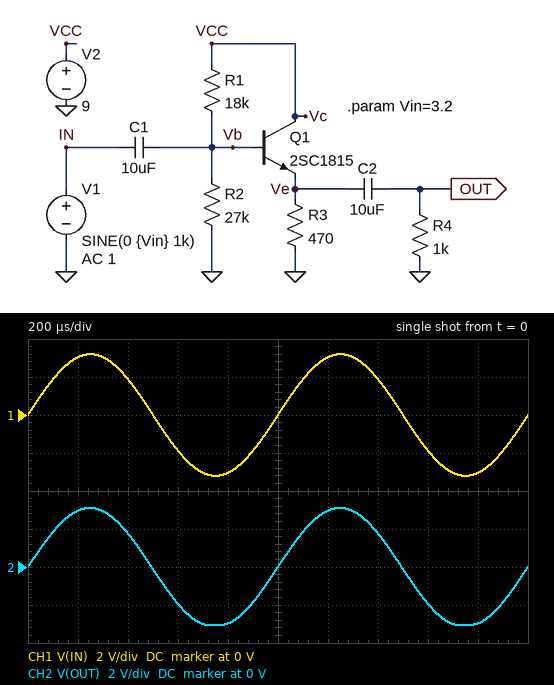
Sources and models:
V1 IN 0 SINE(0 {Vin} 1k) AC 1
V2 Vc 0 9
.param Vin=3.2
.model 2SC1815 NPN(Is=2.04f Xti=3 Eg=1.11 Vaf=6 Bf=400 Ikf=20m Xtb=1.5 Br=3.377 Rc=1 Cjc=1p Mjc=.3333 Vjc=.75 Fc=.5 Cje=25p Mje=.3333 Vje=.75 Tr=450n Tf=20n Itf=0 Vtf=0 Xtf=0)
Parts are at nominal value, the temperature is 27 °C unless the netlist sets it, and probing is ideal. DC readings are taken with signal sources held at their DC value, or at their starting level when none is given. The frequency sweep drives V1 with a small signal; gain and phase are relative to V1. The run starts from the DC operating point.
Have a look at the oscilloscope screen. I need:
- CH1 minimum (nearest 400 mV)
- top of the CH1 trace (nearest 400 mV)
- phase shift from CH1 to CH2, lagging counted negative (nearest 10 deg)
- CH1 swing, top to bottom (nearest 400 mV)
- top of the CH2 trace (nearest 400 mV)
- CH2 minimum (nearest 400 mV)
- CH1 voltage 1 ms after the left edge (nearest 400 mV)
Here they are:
-3.2 V
3.2 V
0 deg
6.4 V
3.2 V
-3.2 V
0 V
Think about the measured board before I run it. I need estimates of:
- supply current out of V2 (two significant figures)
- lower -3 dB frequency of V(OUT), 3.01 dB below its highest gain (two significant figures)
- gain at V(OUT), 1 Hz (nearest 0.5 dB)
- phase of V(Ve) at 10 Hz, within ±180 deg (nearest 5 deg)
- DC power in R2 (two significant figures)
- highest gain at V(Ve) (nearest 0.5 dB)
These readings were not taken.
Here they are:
9.7 mA
16 Hz
-29.5 dB
10 deg
1.0 mW
0 dB
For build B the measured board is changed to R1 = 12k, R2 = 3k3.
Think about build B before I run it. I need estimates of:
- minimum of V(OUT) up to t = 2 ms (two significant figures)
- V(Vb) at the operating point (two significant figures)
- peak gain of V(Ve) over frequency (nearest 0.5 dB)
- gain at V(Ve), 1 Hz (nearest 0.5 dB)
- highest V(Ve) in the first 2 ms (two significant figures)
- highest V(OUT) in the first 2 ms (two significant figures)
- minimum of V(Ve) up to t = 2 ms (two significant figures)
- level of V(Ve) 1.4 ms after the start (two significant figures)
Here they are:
-940 mV
1.9 V
-0.5 dB
-16.0 dB
4.4 V
3.1 V
410 mV
3.0 V
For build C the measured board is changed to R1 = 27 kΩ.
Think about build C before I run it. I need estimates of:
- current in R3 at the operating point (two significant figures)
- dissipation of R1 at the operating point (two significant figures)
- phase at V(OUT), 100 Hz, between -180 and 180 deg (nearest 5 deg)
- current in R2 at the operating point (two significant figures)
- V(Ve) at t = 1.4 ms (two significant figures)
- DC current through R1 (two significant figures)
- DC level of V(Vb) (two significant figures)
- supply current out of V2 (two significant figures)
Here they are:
7.6 mA
810 µW
10 deg
160 µA
5.4 V
170 µA
4.3 V
7.8 mA
